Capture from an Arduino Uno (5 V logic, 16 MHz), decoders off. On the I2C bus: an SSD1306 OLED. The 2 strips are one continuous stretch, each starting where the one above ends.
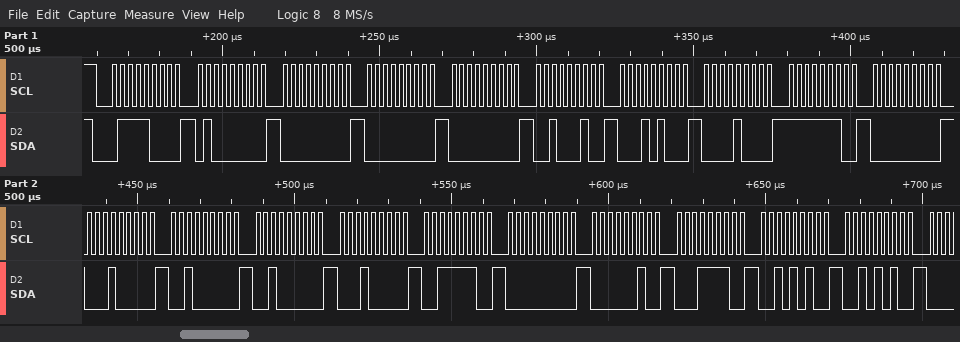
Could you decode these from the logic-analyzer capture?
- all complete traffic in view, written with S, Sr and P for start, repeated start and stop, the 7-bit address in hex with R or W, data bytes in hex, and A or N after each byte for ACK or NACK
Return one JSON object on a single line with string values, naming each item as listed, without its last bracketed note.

{"all complete traffic in view, written with S, Sr and P for start, repeated start and stop, the 7-bit address in hex with R or W, data bytes in hex, and A or N after each byte for ACK or NACK": "S 3CW A 40 A 00 A 00 A 00 A 22 A 14 A 08 A FE A 00 A 10 A 20 A 20 A 10 A 3E A 00 A 02 A 1E A 2A A 2A A"}
